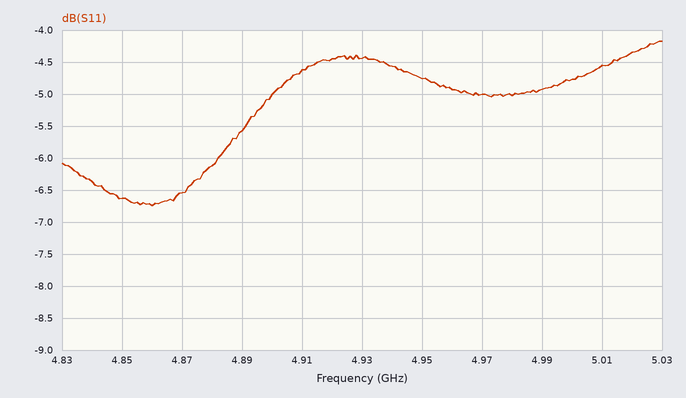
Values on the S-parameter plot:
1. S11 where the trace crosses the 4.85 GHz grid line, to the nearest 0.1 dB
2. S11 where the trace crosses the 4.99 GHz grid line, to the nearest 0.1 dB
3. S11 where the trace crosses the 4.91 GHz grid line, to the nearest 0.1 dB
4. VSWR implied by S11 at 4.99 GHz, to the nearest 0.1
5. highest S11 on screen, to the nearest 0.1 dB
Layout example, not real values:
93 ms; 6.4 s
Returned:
-6.6 dB; -4.9 dB; -4.6 dB; 3.6; -4.2 dB
